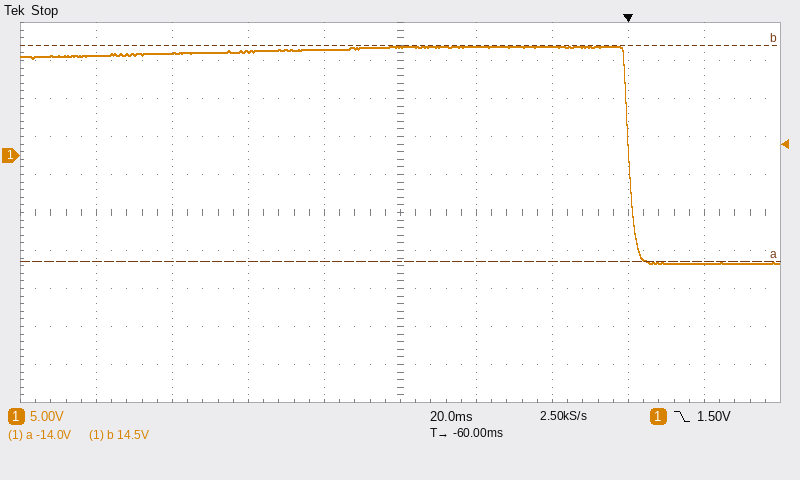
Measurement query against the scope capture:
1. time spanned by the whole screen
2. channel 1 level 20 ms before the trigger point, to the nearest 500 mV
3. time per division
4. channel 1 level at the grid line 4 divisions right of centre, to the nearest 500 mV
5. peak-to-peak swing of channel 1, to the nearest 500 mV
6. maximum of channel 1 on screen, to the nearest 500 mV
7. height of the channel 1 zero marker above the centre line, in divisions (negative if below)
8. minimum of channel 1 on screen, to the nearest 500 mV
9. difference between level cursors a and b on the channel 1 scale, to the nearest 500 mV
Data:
200 ms
14.5 V
20 ms
-14.0 V
28.5 V
14.5 V
+1.5 div
-14.0 V
28.5 V
